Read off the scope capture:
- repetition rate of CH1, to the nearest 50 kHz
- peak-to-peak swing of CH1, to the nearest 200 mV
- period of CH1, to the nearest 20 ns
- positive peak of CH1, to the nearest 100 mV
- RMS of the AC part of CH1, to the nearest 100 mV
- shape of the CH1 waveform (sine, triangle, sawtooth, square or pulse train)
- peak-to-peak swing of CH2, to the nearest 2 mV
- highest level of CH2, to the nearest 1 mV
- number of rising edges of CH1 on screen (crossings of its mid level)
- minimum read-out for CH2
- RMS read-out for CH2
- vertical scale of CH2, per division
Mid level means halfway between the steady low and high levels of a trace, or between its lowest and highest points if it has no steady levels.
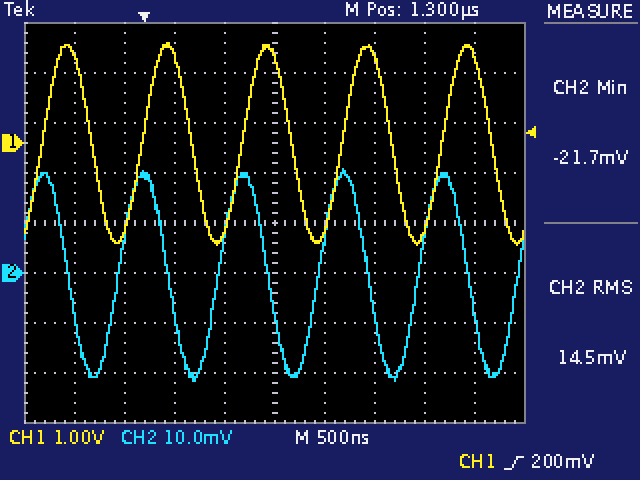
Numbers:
1.00 MHz
4.0 V
1.00 µs
2.0 V
1.4 V
sine
42 mV
21 mV
5
-21.7 mV
14.5 mV
10 mV
